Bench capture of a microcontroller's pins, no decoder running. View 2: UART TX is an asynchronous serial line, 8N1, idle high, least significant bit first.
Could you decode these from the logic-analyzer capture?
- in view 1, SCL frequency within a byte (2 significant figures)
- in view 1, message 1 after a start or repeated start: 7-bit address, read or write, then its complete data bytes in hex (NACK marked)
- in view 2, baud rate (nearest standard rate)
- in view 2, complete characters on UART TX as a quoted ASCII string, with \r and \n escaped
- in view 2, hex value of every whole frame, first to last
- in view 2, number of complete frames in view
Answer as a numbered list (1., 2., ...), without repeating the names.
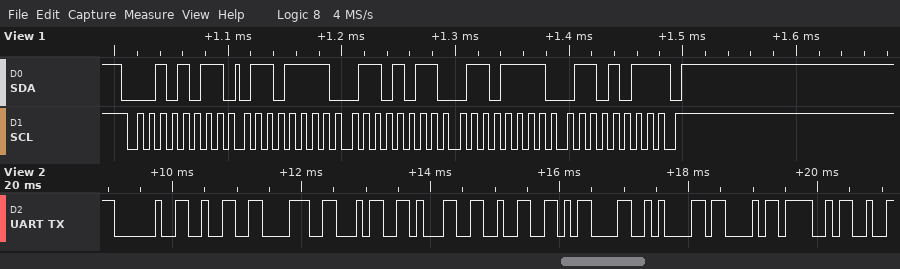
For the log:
1. 100 kHz
2. 0x15 read: 6F 6B 6F 6B NACK
3. 9600 baud
4. " 28412\r\nCO"
5. 20 32 38 34 31 32 0D 0A 43 4F
6. 10
